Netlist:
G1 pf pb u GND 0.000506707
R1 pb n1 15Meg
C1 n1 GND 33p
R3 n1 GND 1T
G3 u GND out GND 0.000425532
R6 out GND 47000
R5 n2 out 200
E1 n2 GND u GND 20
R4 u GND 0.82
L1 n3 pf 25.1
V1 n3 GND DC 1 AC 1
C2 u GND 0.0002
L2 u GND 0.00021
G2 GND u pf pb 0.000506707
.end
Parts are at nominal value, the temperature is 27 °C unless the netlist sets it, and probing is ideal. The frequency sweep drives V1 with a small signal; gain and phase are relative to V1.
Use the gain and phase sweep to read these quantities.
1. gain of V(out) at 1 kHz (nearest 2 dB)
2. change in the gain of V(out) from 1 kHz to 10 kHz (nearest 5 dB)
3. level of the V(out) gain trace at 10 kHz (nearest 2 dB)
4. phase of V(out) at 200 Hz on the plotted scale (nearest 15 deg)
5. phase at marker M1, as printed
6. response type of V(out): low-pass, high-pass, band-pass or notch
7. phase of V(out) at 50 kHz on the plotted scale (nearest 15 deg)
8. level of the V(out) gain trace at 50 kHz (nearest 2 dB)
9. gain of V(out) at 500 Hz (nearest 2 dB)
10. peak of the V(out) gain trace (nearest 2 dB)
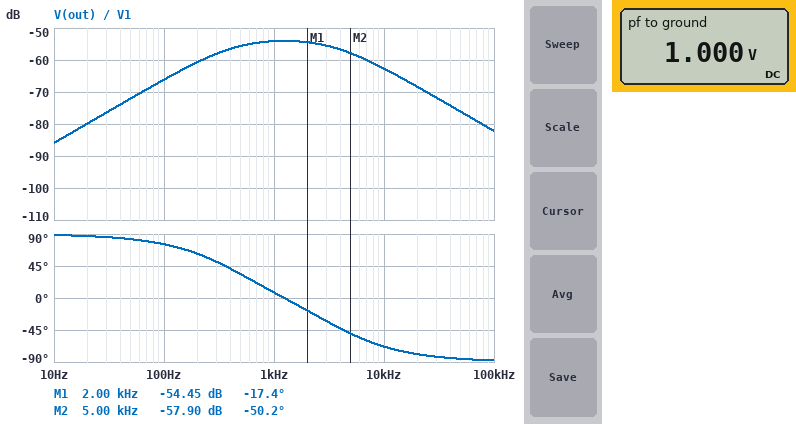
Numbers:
-54 dB
-10 dB
-62 dB
60 deg
-17.4 deg
band-pass
-90 deg
-76 dB
-56 dB
-54 dB
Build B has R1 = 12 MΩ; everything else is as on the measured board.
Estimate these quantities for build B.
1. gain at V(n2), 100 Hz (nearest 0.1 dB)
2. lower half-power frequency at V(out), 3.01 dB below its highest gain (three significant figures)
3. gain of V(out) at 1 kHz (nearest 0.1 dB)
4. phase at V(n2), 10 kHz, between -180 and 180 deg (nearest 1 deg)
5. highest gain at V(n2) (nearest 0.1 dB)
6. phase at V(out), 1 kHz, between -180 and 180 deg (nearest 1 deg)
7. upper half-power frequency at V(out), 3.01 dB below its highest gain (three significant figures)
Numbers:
-66.0 dB
412 Hz
-52.7 dB
-71 deg
-52.6 dB
9 deg
3.73 kHz
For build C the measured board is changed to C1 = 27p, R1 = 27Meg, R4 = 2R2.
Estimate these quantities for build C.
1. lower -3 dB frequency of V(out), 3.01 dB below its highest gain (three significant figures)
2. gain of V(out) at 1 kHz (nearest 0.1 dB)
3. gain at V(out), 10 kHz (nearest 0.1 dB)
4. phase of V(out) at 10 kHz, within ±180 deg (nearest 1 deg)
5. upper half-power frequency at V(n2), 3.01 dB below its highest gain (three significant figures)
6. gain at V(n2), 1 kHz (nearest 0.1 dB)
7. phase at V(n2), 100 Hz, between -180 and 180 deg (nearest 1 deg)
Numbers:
292 Hz
-57.4 dB
-63.3 dB
-60 deg
5.99 kHz
-57.3 dB
72 deg
